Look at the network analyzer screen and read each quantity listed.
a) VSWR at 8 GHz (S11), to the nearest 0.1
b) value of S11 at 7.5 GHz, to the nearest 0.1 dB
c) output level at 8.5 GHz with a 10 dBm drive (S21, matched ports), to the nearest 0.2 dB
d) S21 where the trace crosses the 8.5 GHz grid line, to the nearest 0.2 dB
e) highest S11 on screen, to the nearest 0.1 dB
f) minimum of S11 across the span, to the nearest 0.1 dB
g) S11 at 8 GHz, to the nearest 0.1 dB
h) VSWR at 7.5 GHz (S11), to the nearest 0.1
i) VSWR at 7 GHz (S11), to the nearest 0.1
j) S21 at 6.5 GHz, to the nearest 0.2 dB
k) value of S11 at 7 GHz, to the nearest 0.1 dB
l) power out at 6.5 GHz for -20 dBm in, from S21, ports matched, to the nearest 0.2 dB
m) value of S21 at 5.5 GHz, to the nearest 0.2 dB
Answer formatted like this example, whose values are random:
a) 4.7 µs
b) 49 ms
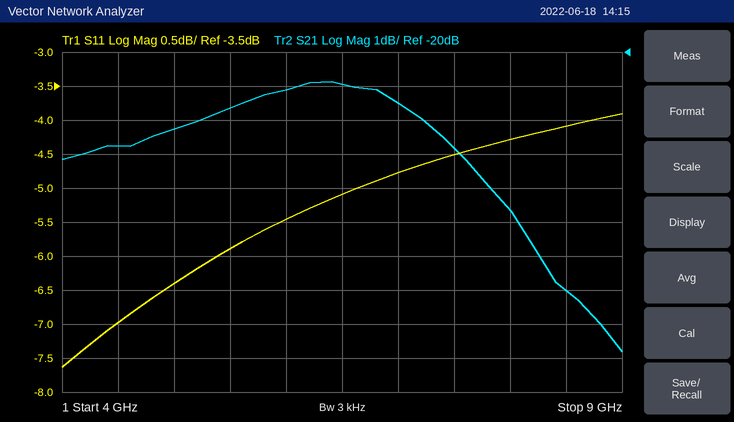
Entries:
a) 4.1
b) -4.5 dB
c) -17.0 dBm
d) -27.0 dB
e) -3.9 dB
f) -7.6 dB
g) -4.3 dB
h) 3.9
i) 3.7
j) -21.0 dB
k) -4.8 dB
l) -41.0 dBm
m) -21.6 dB
